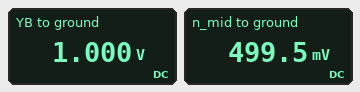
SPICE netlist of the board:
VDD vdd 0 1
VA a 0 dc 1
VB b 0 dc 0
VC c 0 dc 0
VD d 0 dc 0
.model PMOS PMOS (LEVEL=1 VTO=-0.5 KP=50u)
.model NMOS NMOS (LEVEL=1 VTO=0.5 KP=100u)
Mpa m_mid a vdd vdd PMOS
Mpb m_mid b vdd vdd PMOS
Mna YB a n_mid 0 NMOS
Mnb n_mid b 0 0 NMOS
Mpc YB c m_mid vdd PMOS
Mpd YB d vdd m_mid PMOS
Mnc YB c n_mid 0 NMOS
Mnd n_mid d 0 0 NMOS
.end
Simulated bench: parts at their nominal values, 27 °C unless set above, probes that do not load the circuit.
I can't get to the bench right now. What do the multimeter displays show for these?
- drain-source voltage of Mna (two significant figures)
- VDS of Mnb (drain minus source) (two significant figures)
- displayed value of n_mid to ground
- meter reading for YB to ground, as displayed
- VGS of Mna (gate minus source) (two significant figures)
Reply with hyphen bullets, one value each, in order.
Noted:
- 500 mV
- 500 mV
- 499.5 mV
- 1.000 V
- 500 mV
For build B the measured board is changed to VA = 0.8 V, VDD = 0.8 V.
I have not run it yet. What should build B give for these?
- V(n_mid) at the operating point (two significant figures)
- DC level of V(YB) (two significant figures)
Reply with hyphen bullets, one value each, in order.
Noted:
- 300 mV
- 800 mV
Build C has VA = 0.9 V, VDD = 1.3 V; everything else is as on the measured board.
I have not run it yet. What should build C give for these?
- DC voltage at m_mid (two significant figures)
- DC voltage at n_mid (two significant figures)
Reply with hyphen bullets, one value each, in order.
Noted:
- 1.3 V
- 400 mV
